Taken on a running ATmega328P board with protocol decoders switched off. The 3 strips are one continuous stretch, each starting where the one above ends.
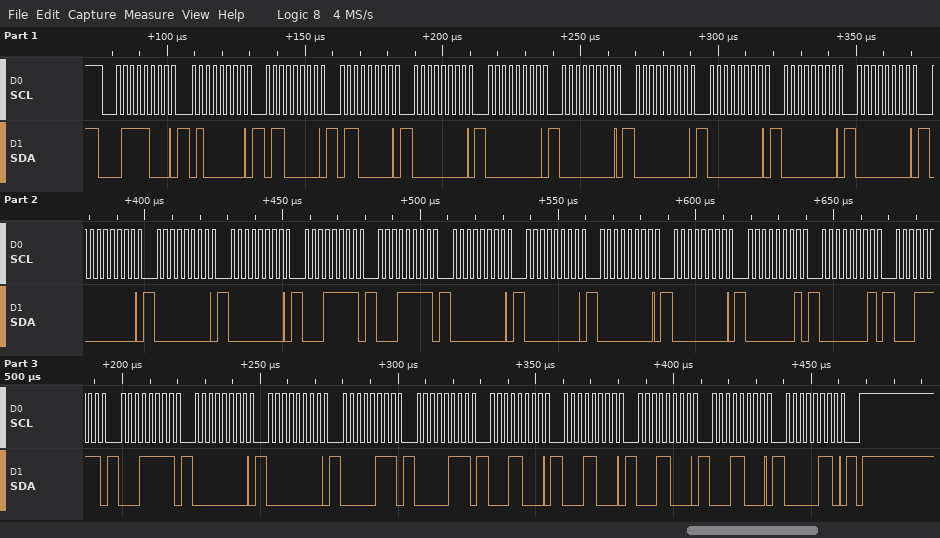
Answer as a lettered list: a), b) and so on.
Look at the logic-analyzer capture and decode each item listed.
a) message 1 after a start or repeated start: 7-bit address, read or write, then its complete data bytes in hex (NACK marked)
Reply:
a) 0x3C write: 40 60 60 00 00 00 00 00 00 00 00 00 00 1F 1F 00 00 00 00 01 01 1F 1F 00 00 07 07 18 18 18 18 06
